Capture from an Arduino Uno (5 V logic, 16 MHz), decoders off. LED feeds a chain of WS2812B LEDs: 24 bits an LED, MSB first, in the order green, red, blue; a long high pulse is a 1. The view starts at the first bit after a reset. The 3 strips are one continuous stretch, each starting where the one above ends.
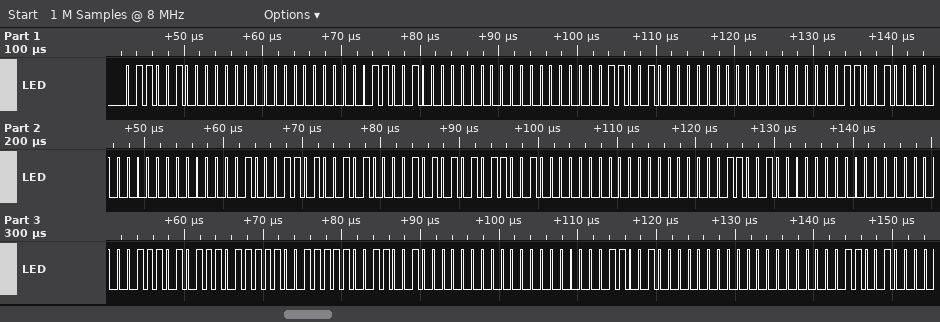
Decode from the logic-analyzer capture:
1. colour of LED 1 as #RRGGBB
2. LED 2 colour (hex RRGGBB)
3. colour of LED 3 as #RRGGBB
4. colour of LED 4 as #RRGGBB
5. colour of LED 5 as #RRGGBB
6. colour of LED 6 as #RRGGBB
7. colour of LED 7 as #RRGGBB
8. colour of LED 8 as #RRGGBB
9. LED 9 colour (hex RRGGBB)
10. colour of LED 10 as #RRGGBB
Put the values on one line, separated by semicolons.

#006400; #006400; #006400; #006400; #288D55; #006400; #006400; #DF753E; #006400; #006400
